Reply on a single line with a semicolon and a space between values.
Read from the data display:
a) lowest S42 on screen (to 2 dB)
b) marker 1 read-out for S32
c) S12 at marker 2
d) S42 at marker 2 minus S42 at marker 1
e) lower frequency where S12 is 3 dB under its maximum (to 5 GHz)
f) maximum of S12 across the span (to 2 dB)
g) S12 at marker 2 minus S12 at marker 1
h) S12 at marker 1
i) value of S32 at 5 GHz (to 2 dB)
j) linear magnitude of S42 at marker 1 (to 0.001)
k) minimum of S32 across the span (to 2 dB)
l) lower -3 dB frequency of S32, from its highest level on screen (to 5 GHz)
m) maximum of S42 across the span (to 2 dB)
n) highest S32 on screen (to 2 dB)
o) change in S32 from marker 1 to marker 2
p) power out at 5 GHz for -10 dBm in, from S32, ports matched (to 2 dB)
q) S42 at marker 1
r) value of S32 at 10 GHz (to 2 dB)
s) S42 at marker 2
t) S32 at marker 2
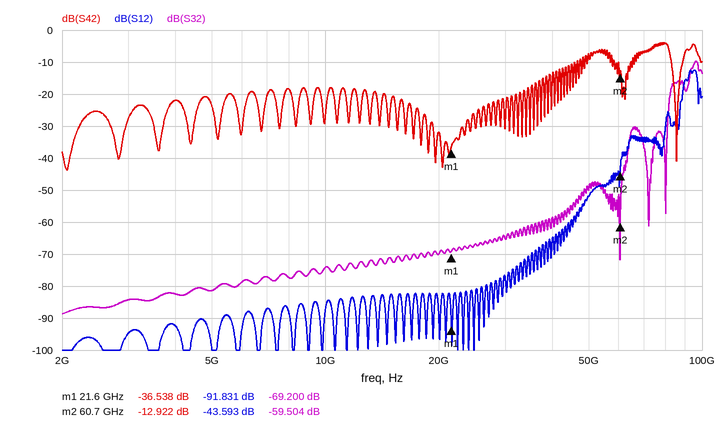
-44 dB; -69.200 dB; -43.593 dB; 23.616 dB; 90 GHz; -12 dB; 48.238 dB; -91.831 dB; -82 dB; 0.015; -88 dB; 95 GHz; -4 dB; -10 dB; 9.696 dB; -92 dBm; -36.538 dB; -74 dB; -12.922 dB; -59.504 dB
